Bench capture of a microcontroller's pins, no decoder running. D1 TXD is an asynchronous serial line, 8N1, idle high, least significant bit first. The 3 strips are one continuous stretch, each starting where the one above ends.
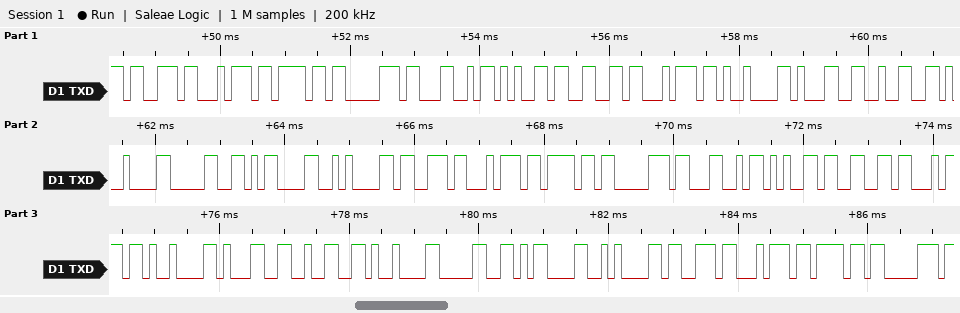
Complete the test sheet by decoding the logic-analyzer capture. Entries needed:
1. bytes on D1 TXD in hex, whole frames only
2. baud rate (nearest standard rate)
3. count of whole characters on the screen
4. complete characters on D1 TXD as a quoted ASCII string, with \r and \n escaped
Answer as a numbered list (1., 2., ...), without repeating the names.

1. 73 74 6F 70 4C 65 66 74 09 31 32 09 30 0D 0A 73 74 6F 70 4C 65 66 74 09 31 32 09 30 0D 0A 73 74 6F 70
2. 9600 baud
3. 34
4. "stopLeft\t12\t0\r\nstopLeft\t12\t0\r\nstop"
